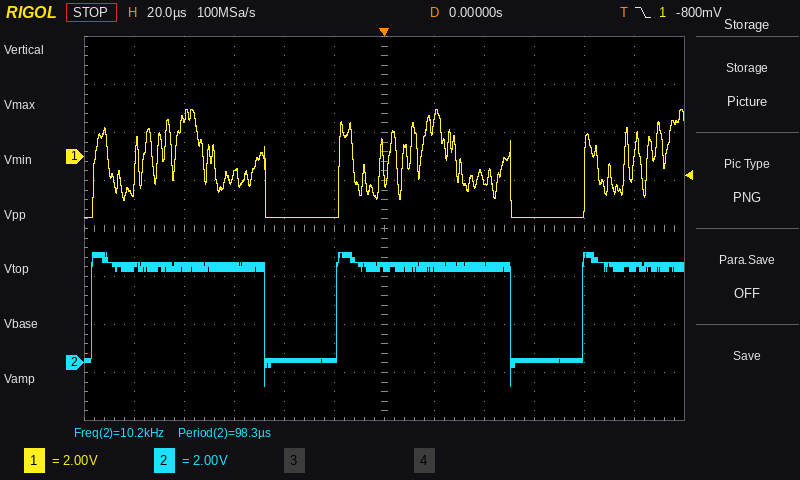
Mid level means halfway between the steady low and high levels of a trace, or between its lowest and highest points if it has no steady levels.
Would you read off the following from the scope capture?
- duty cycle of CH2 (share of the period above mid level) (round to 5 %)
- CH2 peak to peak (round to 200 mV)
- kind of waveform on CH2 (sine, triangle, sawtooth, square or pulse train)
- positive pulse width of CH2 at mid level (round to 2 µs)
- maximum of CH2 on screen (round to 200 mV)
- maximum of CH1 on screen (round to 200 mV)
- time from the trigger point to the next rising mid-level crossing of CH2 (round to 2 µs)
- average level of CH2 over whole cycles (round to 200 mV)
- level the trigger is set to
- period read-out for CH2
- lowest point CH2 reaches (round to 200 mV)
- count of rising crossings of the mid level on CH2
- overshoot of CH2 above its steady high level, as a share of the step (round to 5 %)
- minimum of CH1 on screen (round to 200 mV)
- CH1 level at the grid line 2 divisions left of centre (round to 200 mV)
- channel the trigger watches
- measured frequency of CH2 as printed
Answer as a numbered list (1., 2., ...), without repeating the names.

1. 70 %
2. 5.6 V
3. pulse train
4. 70 µs
5. 4.6 V
6. 2.0 V
7. 80 µs
8. 3.0 V
9. -800 mV
10. 98.3 µs
11. -1.0 V
12. 3
13. 15 %
14. -2.6 V
15. -2.6 V
16. CH1
17. 10.2 kHz
